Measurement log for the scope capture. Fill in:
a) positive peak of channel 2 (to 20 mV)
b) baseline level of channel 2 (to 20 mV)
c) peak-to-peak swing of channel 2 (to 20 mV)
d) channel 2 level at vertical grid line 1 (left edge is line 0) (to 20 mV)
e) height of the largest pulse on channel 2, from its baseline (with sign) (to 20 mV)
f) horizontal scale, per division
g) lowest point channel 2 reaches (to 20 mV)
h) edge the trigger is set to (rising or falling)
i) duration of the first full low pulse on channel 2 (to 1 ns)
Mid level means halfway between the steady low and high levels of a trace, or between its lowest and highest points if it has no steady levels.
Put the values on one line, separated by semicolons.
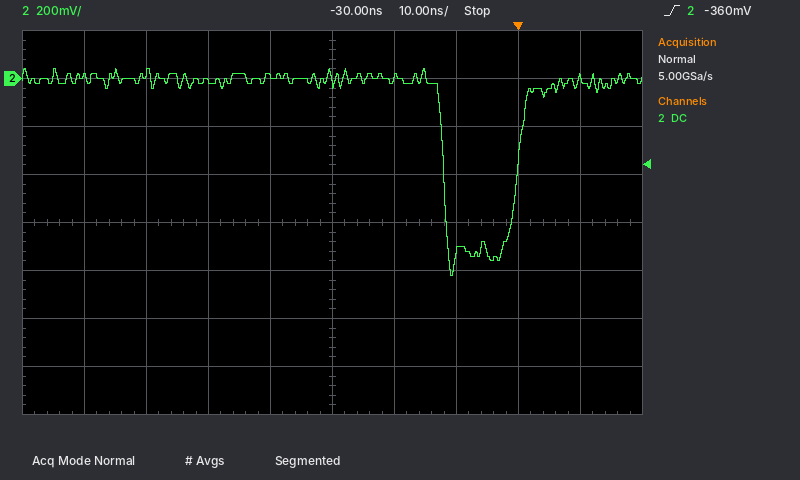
40 mV; 0 mV; 860 mV; 0 mV; -820 mV; 10 ns; -820 mV; rising; 12 ns
